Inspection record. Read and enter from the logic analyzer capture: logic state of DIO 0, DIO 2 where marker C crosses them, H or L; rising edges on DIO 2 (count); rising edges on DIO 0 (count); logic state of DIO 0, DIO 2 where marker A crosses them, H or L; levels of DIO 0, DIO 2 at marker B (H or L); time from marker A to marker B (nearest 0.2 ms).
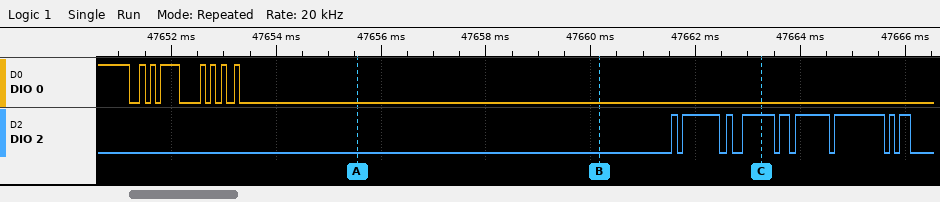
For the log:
DIO 0=L, DIO 2=H
9
7
DIO 0=L, DIO 2=L
DIO 0=L, DIO 2=L
4.6 ms
